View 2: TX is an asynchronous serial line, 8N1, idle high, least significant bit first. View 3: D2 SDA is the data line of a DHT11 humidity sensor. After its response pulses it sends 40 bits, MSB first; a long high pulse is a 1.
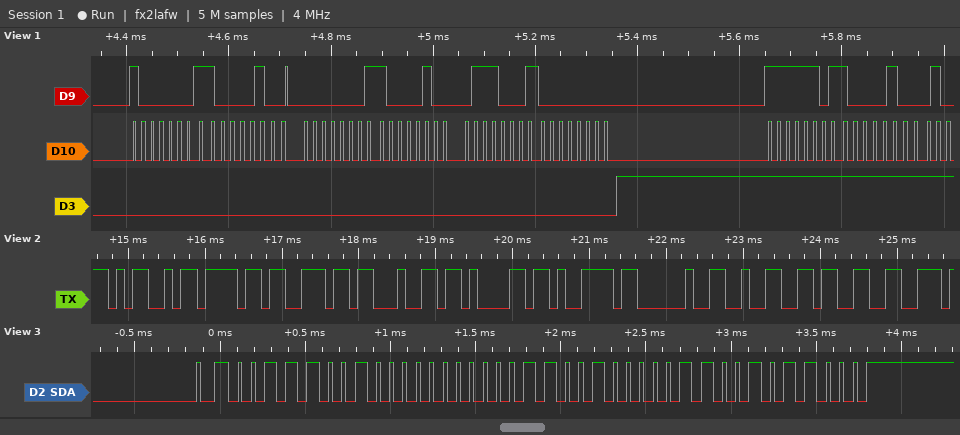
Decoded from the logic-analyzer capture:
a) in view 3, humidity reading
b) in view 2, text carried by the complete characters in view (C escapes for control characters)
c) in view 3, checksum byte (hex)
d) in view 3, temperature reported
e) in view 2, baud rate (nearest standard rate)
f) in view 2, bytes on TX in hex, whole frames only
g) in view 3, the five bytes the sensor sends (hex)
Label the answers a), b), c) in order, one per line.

a) 57 %
b) "Monday 23"
c) 0x58
d) 25.6 °C
e) 9600 baud
f) 4D 6F 6E 64 61 79 20 32 33
g) 39 00 19 06 58
